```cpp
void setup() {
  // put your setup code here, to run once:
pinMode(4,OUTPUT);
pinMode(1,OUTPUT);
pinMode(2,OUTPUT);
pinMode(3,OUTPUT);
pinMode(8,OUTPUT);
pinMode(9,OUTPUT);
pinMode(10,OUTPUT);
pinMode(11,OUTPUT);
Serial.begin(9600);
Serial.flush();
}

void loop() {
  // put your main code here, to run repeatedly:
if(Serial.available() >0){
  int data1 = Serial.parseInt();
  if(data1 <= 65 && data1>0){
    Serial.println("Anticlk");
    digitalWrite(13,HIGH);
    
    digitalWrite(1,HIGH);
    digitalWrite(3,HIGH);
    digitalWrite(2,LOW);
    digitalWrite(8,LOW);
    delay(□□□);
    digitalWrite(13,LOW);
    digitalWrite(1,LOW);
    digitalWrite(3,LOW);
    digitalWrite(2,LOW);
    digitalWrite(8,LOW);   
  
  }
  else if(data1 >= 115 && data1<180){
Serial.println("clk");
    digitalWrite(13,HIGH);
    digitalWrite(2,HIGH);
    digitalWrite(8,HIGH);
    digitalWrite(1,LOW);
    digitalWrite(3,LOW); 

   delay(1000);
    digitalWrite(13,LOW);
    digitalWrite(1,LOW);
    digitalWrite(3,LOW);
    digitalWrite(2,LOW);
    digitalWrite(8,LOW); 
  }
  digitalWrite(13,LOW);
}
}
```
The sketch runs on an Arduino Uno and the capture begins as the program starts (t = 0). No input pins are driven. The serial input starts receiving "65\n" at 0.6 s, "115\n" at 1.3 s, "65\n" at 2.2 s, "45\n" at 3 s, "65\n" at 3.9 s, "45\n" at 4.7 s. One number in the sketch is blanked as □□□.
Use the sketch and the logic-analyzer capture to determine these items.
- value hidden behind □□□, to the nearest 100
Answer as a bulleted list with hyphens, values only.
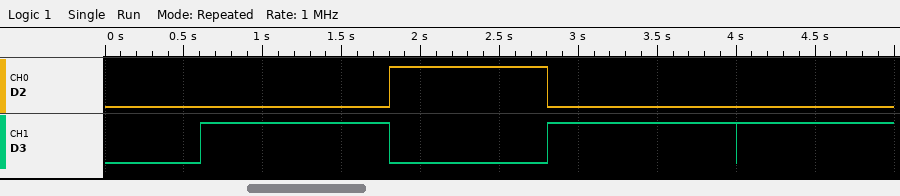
- 1200
